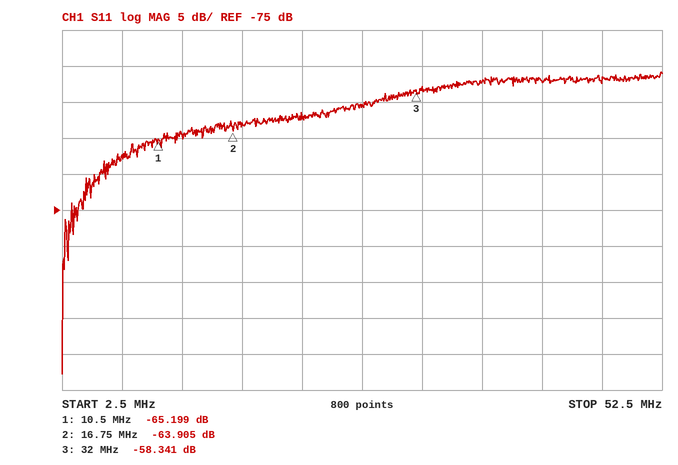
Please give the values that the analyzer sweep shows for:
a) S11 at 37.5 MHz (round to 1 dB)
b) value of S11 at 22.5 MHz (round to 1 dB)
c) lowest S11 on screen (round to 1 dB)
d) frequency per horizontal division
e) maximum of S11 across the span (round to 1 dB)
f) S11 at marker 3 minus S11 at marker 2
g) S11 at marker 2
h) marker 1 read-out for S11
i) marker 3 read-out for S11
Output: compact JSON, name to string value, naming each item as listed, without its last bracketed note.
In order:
{"S11 at 37.5 MHz": "-57 dB", "value of S11 at 22.5 MHz": "-62 dB", "lowest S11 on screen": "-98 dB", "frequency per horizontal division": "5 MHz", "maximum of S11 across the span": "-56 dB", "S11 at marker 3 minus S11 at marker 2": "5.564 dB", "S11 at marker 2": "-63.905 dB", "marker 1 read-out for S11": "-65.199 dB", "marker 3 read-out for S11": "-58.341 dB"}
